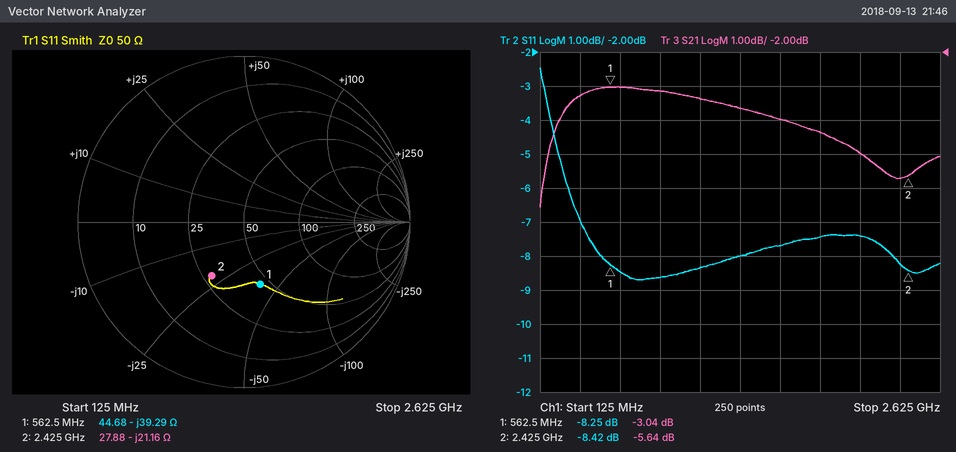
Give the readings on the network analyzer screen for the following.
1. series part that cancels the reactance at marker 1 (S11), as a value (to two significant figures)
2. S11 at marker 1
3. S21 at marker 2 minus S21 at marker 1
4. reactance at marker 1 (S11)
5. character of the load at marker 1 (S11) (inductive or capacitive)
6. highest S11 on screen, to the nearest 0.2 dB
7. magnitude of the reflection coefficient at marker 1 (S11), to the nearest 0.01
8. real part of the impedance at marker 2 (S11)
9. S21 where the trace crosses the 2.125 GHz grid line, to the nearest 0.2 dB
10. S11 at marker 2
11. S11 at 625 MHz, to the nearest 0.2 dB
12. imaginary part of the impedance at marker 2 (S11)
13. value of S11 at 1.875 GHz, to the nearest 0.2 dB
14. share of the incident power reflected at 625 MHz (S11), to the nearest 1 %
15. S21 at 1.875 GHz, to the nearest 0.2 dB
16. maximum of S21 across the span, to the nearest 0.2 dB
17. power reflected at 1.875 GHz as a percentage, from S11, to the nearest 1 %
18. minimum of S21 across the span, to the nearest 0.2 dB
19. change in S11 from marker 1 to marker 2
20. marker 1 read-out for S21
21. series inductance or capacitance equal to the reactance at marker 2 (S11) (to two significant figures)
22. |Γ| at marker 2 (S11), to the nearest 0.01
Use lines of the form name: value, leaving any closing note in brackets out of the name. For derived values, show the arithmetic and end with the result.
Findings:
series part that cancels the reactance at marker 1 (S11), as a value: L = 39.29 Ω/(2π × 562.5 MHz) ≈ 11 nH
S11 at marker 1: -8.25 dB
S21 at marker 2 minus S21 at marker 1: -5.64 − (-3.04) = -2.60 dB
reactance at marker 1: -39.29 Ω
character of the load at marker 1 (S11): capacitive
highest S11 on screen, to the nearest 0.2 dB: -2.4 dB
magnitude of the reflection coefficient at marker 1 (S11), to the nearest 0.01: 0.39
real part of the impedance at marker 2: 27.88 Ω
S21 where the trace crosses the 2.125 GHz grid line, to the nearest 0.2 dB: -5.0 dB
S11 at marker 2: -8.42 dB
S11 at 625 MHz, to the nearest 0.2 dB: -8.4 dB
imaginary part of the impedance at marker 2: -21.16 Ω
value of S11 at 1.875 GHz, to the nearest 0.2 dB: -7.4 dB
share of the incident power reflected at 625 MHz (S11), to the nearest 1 %: 10^(-8.4/10) ≈ 14 %
S21 at 1.875 GHz, to the nearest 0.2 dB: -4.4 dB
maximum of S21 across the span, to the nearest 0.2 dB: -3.0 dB
power reflected at 1.875 GHz as a percentage, from S11, to the nearest 1 %: 10^(-7.4/10) ≈ 18 %
minimum of S21 across the span, to the nearest 0.2 dB: -6.6 dB
change in S11 from marker 1 to marker 2: -8.42 − (-8.25) = -0.17 dB
marker 1 read-out for S21: -3.04 dB
series inductance or capacitance equal to the reactance at marker 2 (S11): C = 1/(2π × 2.425 GHz × 21.16 Ω) ≈ 3.1 pF
|Γ| at marker 2 (S11), to the nearest 0.01: 0.38
